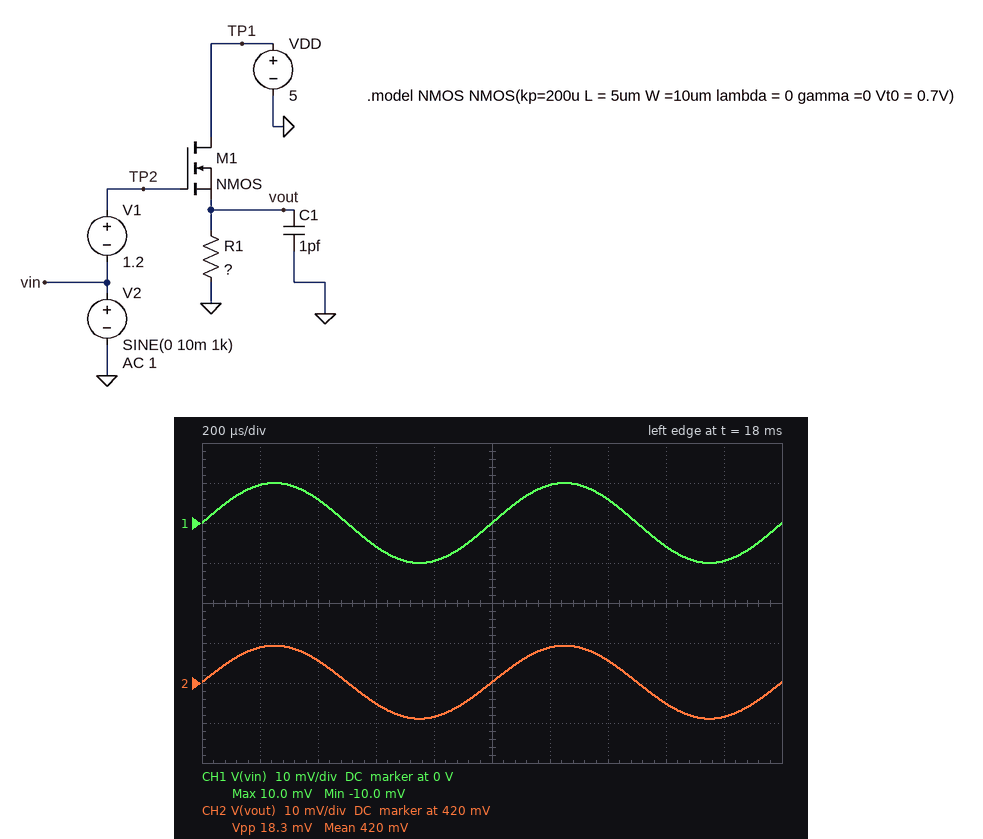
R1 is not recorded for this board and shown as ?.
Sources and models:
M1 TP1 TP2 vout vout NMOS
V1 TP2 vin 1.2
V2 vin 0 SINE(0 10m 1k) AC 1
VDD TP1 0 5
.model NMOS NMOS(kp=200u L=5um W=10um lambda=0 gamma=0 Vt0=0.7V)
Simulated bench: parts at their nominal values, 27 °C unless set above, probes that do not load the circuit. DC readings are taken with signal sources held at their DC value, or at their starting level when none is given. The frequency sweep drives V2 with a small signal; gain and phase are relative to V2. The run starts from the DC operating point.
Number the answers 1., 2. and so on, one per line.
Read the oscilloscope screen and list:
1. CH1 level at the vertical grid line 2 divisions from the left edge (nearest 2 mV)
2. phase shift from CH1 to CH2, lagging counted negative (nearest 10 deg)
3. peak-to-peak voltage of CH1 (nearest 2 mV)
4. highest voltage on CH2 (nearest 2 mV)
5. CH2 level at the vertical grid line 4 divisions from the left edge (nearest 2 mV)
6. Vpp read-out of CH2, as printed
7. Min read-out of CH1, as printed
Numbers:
1. 6 mV
2. 0 deg
3. 20 mV
4. 430 mV
5. 412 mV
6. 18.3 mV
7. -10.0 mV
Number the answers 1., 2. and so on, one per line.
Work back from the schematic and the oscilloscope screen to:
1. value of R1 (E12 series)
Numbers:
1. 330 kΩ
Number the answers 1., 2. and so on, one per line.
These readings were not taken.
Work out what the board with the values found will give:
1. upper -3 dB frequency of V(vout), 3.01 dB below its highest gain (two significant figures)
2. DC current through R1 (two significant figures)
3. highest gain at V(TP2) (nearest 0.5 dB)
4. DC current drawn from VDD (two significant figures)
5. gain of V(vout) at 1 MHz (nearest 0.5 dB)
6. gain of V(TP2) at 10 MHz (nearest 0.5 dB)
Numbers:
1. 5.6 MHz
2. 1.3 µA
3. 0 dB
4. 1.3 µA
5. -1.0 dB
6. 0 dB
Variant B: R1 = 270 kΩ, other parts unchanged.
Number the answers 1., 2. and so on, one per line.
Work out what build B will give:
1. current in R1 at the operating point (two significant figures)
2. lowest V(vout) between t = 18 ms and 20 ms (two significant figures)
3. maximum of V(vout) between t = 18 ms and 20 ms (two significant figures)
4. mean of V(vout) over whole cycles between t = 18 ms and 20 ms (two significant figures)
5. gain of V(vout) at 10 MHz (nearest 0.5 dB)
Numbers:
1. 1.5 µA
2. 400 mV
3. 420 mV
4. 410 mV
5. -6.5 dB
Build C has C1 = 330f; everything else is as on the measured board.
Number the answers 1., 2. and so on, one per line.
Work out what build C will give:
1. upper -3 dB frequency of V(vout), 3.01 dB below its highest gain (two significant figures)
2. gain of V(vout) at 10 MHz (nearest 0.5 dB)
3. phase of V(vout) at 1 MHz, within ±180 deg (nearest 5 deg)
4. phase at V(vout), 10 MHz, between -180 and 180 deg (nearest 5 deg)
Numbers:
1. 17 MHz
2. -2.0 dB
3. -5 deg
4. -30 deg
